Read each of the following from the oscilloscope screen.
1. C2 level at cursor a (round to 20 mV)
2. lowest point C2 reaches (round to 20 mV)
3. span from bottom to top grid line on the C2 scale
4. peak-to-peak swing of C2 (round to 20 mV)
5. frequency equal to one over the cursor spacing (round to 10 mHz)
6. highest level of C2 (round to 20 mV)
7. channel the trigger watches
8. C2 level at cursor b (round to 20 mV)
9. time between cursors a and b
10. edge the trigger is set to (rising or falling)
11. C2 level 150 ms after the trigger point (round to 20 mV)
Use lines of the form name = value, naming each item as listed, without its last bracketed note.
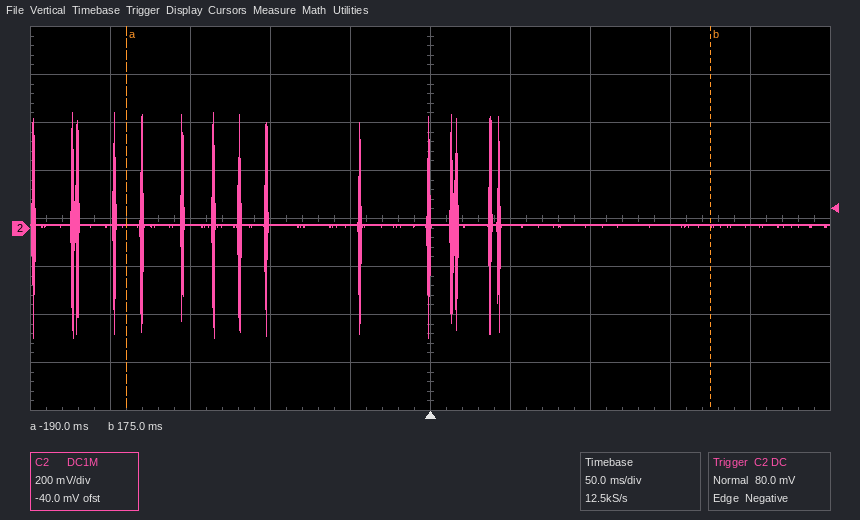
C2 level at cursor a = 20 mV
lowest point C2 reaches = -460 mV
span from bottom to top grid line on the C2 scale = 1.6 V
peak-to-peak swing of C2 = 940 mV
frequency equal to one over the cursor spacing = 2.74 Hz
highest level of C2 = 480 mV
channel the trigger watches = C2
C2 level at cursor b = 20 mV
time between cursors a and b = 365 ms
edge the trigger is set to = falling
C2 level 150 ms after the trigger point = 20 mV
